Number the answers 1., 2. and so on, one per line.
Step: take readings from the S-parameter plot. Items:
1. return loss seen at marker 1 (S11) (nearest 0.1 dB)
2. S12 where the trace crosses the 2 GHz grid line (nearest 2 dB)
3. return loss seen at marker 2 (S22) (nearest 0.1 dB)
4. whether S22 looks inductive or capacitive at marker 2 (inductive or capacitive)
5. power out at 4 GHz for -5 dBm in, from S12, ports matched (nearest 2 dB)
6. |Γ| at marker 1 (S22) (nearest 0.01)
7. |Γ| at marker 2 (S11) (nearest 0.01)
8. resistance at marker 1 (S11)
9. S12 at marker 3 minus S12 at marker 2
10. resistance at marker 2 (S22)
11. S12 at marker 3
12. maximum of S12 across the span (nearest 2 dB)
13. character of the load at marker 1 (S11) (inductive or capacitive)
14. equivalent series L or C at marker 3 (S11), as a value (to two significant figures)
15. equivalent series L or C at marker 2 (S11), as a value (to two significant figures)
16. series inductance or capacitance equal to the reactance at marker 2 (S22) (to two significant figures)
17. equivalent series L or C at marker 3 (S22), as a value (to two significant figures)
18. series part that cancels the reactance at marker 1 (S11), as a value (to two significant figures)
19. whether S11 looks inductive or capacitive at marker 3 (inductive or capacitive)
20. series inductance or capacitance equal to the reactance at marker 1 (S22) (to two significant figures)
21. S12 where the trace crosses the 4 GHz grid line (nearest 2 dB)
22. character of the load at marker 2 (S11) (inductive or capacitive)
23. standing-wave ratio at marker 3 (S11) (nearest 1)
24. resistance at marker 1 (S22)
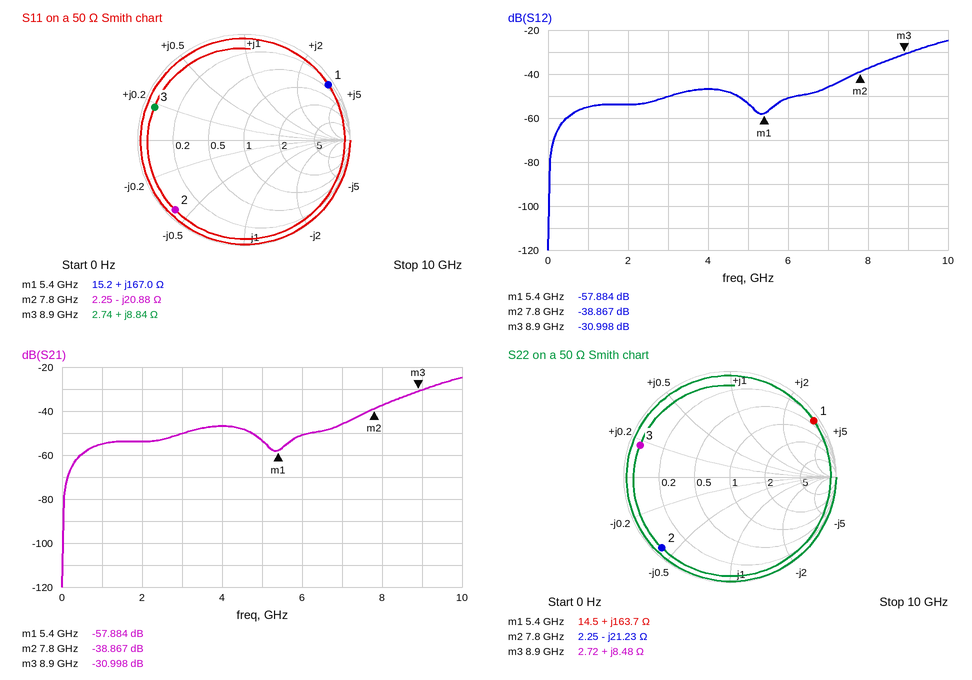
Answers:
1. 0.4 dB
2. -54 dB
3. 0.7 dB
4. capacitive
5. -52 dBm
6. 0.95
7. 0.93
8. 15.2 Ω
9. 7.869 dB
10. 2.25 Ω
11. -30.998 dB
12. -24 dB
13. inductive
14. 160 pH
15. 980 fF
16. 960 fF
17. 150 pH
18. 180 fF
19. inductive
20. 4.8 nH
21. -46 dB
22. capacitive
23. 19
24. 14.5 Ω
